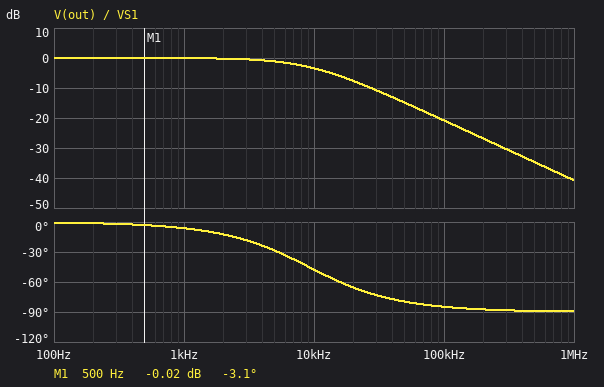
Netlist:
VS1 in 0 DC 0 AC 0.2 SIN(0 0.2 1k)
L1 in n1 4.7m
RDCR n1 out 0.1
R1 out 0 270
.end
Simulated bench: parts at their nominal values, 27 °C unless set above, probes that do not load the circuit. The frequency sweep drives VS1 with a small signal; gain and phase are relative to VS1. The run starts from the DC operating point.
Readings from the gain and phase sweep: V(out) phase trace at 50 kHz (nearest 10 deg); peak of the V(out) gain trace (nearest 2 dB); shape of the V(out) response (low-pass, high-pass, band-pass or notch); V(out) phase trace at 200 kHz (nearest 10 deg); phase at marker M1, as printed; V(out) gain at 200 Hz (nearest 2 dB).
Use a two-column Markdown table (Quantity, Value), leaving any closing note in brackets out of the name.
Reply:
| Quantity | Value |
|---|---|
| V(out) phase trace at 50 kHz | -80 deg |
| peak of the V(out) gain trace | 0 dB |
| shape of the V(out) response | low-pass |
| V(out) phase trace at 200 kHz | -90 deg |
| phase at marker M1, as printed | -3.1 deg |
| V(out) gain at 200 Hz | 0 dB |
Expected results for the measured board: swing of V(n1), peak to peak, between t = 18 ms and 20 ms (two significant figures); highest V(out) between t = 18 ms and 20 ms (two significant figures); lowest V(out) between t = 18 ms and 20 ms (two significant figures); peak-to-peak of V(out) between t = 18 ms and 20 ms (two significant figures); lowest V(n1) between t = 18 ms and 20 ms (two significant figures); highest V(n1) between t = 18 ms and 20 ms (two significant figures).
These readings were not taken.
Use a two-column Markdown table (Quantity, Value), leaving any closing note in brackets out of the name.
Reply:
| Quantity | Value |
|---|---|
| swing of V(n1), peak to peak, between t = 18 ms and 20 ms | 400 mV |
| highest V(out) between t = 18 ms and 20 ms | 200 mV |
| lowest V(out) between t = 18 ms and 20 ms | -200 mV |
| peak-to-peak of V(out) between t = 18 ms and 20 ms | 400 mV |
| lowest V(n1) between t = 18 ms and 20 ms | -200 mV |
| highest V(n1) between t = 18 ms and 20 ms | 200 mV |
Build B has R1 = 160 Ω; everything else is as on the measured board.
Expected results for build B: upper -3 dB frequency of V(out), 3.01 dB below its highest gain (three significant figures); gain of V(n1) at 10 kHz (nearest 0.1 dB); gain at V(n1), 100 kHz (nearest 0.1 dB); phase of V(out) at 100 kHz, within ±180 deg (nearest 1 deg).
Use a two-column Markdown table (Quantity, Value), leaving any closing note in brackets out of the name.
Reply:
| Quantity | Value |
|---|---|
| upper -3 dB frequency of V(out), 3.01 dB below its highest gain | 5.42 kHz |
| gain of V(n1) at 10 kHz | -6.4 dB |
| gain at V(n1), 100 kHz | -25.3 dB |
| phase of V(out) at 100 kHz, within ±180 deg | -87 deg |
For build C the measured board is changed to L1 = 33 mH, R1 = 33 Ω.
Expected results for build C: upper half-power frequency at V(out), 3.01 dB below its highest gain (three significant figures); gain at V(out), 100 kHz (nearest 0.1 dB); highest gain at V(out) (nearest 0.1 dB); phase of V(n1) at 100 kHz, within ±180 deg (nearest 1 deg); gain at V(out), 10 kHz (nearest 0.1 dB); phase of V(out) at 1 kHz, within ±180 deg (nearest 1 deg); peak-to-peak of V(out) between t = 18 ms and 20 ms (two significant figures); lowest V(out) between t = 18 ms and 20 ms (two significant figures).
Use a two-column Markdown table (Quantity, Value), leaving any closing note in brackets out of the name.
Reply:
| Quantity | Value |
|---|---|
| upper half-power frequency at V(out), 3.01 dB below its highest gain | 160 Hz |
| gain at V(out), 100 kHz | -56.0 dB |
| highest gain at V(out) | 0 dB |
| phase of V(n1) at 100 kHz, within ±180 deg | -90 deg |
| gain at V(out), 10 kHz | -36.0 dB |
| phase of V(out) at 1 kHz, within ±180 deg | -81 deg |
| peak-to-peak of V(out) between t = 18 ms and 20 ms | 63 mV |
| lowest V(out) between t = 18 ms and 20 ms | -31 mV |
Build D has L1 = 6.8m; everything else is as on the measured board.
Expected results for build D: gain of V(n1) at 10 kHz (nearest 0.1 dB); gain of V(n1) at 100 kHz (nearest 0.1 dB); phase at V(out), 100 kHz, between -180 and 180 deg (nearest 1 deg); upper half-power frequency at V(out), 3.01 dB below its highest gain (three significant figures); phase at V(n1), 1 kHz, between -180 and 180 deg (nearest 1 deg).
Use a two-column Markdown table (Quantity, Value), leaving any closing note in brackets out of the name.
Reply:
| Quantity | Value |
|---|---|
| gain of V(n1) at 10 kHz | -5.4 dB |
| gain of V(n1) at 100 kHz | -24.0 dB |
| phase at V(out), 100 kHz, between -180 and 180 deg | -86 deg |
| upper half-power frequency at V(out), 3.01 dB below its highest gain | 6.32 kHz |
| phase at V(n1), 1 kHz, between -180 and 180 deg | -9 deg |
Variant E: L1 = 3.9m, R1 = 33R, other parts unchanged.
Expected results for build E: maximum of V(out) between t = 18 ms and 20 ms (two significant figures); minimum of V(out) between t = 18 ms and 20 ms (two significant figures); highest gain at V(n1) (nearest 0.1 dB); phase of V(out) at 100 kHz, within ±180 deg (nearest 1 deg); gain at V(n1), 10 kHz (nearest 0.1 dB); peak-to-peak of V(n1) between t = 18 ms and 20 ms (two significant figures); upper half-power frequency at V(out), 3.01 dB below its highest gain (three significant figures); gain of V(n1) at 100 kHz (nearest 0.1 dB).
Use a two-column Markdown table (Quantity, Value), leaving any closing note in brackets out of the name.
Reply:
| Quantity | Value |
|---|---|
| maximum of V(out) between t = 18 ms and 20 ms | 160 mV |
| minimum of V(out) between t = 18 ms and 20 ms | -160 mV |
| highest gain at V(n1) | 0 dB |
| phase of V(out) at 100 kHz, within ±180 deg | -89 deg |
| gain at V(n1), 10 kHz | -17.5 dB |
| peak-to-peak of V(n1) between t = 18 ms and 20 ms | 320 mV |
| upper half-power frequency at V(out), 3.01 dB below its highest gain | 1.35 kHz |
| gain of V(n1) at 100 kHz | -37.4 dB |
